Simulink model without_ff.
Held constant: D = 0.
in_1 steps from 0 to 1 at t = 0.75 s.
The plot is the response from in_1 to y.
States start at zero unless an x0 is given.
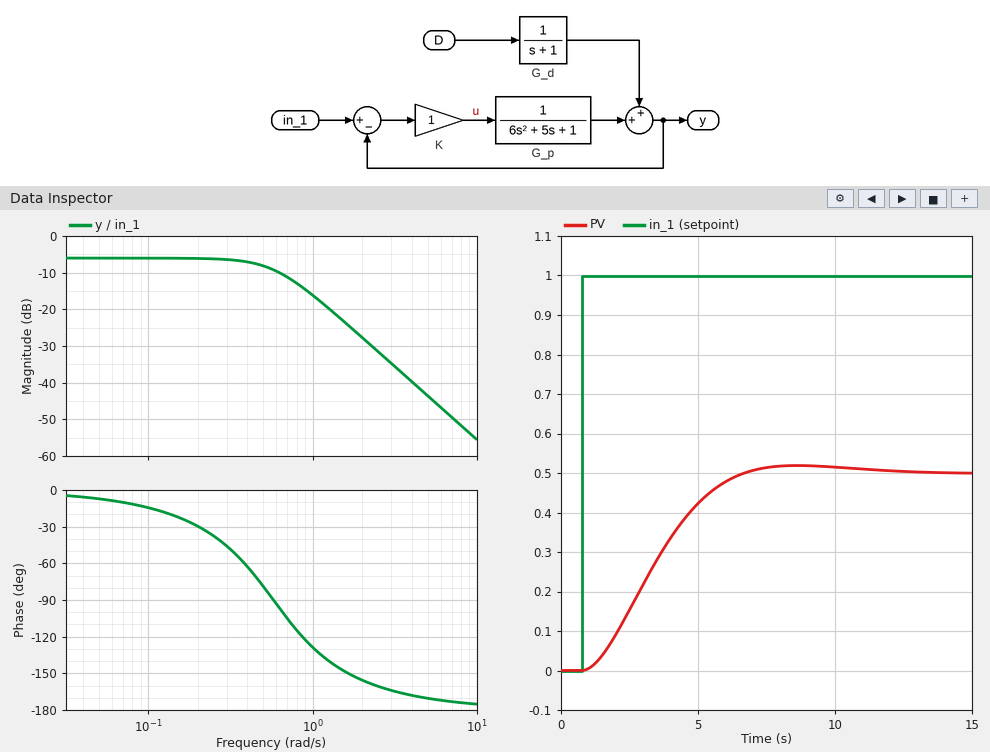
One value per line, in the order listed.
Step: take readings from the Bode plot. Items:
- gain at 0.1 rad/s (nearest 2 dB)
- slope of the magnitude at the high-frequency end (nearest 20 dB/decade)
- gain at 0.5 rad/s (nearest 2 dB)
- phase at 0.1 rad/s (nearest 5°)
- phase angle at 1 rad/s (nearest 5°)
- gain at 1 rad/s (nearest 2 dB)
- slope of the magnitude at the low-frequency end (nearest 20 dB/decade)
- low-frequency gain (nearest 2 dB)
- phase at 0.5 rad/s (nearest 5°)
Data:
-6 dB
-40 dB/decade
-8 dB
-15°
-130°
-16 dB
0 dB/decade
-6 dB
-80°
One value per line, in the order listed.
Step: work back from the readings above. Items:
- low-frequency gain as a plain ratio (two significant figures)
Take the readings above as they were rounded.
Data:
0.50
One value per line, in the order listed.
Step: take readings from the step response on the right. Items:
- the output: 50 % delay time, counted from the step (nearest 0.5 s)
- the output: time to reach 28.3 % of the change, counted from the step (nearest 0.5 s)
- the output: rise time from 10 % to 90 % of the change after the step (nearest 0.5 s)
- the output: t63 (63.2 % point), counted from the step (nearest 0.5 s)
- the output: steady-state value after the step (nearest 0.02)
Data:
2.5 s
1.5 s
4.0 s
3.0 s
0.50
